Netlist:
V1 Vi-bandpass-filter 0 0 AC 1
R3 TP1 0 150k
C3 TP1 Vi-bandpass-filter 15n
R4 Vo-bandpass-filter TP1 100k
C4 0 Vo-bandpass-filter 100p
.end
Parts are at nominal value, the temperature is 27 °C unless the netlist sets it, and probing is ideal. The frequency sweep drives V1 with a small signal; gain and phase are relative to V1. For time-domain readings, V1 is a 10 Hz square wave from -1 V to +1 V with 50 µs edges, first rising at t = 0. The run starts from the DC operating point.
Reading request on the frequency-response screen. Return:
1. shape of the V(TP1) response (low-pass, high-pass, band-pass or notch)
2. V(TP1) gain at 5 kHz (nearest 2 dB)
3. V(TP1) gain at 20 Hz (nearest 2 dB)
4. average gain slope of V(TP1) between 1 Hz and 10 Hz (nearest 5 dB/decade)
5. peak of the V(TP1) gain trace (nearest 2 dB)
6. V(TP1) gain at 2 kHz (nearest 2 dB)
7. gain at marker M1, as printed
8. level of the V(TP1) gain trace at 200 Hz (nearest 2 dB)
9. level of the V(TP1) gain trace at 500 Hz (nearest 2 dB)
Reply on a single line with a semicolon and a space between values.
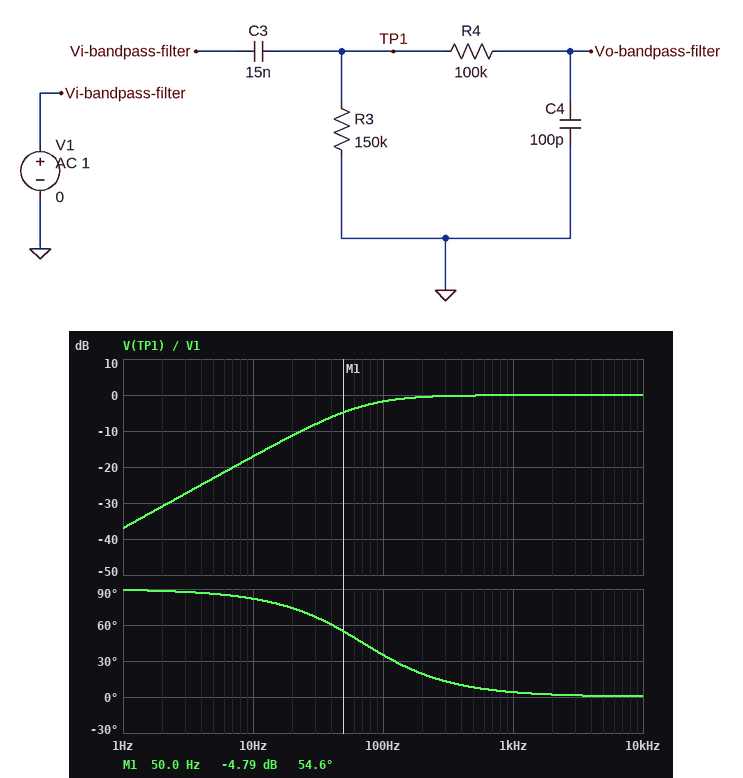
high-pass; 0 dB; -12 dB; 20 dB/decade; 0 dB; 0 dB; -4.79 dB; 0 dB; 0 dB
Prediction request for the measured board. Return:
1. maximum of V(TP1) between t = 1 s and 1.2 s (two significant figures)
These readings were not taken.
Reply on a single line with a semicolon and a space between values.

2.0 V
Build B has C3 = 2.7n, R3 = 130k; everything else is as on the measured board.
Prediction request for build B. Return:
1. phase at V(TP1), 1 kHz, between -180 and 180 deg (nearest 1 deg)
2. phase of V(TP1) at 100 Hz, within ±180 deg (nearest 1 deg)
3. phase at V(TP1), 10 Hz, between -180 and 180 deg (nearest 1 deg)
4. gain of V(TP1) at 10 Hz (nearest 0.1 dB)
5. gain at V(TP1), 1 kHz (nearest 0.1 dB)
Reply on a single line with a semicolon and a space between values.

24 deg; 77 deg; 89 deg; -33.1 dB; -1.1 dB
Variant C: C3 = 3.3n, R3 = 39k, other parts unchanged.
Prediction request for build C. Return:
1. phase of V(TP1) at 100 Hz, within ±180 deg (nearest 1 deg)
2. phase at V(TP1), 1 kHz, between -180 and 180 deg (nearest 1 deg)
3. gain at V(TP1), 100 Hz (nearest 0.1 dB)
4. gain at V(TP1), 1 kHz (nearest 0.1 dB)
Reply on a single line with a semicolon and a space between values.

85 deg; 50 deg; -21.9 dB; -4.1 dB
